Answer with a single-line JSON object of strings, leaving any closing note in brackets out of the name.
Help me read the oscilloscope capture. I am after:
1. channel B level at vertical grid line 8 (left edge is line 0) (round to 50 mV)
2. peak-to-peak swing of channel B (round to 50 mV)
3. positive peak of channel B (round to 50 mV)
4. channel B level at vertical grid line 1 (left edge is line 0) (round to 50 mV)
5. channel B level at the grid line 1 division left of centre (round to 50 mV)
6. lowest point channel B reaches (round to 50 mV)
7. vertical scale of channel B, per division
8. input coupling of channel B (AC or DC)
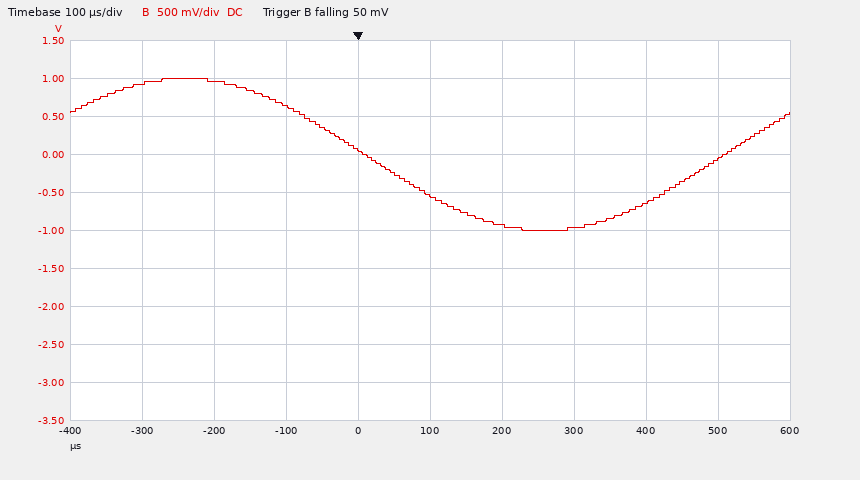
{"channel B level at vertical grid line 8 (left edge is line 0)": "-600 mV", "peak-to-peak swing of channel B": "2.00 V", "positive peak of channel B": "1.00 V", "channel B level at vertical grid line 1 (left edge is line 0)": "950 mV", "channel B level at the grid line 1 division left of centre": "50 mV", "lowest point channel B reaches": "-1.00 V", "vertical scale of channel B, per division": "500 mV", "input coupling of channel B": "DC"}
